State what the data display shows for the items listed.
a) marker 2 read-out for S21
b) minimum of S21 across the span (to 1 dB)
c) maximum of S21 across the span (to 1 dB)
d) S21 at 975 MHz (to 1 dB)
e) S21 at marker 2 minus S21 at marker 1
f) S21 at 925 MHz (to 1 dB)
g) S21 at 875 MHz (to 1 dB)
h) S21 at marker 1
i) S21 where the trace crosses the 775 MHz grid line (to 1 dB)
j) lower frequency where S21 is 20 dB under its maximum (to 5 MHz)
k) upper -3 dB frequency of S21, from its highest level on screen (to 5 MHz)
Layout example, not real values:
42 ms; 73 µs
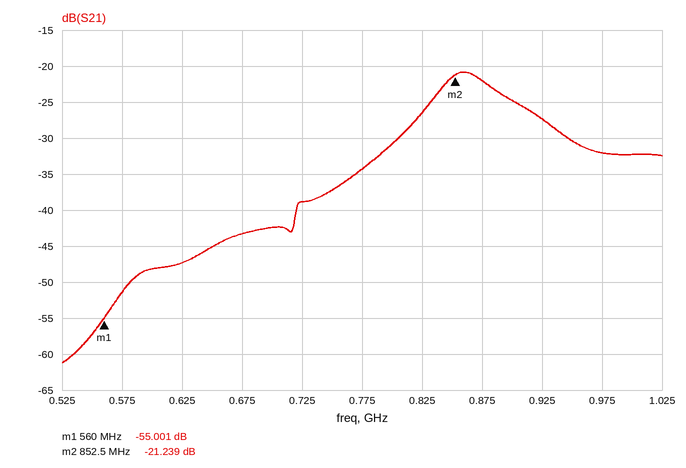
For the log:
-21.239 dB; -61 dB; -21 dB; -32 dB; 33.762 dB; -27 dB; -22 dB; -55.001 dB; -34 dB; 720 MHz; 890 MHz
